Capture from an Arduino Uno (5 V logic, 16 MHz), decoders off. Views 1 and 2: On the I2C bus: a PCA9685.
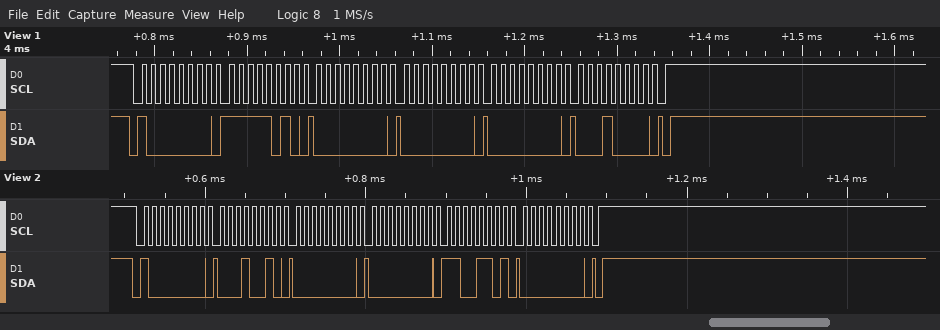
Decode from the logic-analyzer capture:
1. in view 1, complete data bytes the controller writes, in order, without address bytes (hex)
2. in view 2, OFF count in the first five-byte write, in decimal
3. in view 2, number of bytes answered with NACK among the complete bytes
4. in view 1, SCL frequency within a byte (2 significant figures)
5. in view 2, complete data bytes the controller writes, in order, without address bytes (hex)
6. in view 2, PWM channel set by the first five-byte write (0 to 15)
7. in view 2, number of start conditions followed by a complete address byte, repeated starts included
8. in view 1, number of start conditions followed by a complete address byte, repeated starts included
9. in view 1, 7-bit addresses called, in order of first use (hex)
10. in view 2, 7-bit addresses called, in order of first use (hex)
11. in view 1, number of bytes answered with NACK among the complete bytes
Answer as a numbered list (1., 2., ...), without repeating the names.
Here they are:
1. FA 00 00 00 10
2. 205
3. 0
4. 100 kHz
5. 12 00 00 CD 00
6. 3
7. 1
8. 1
9. 0x40
10. 0x40
11. 0
